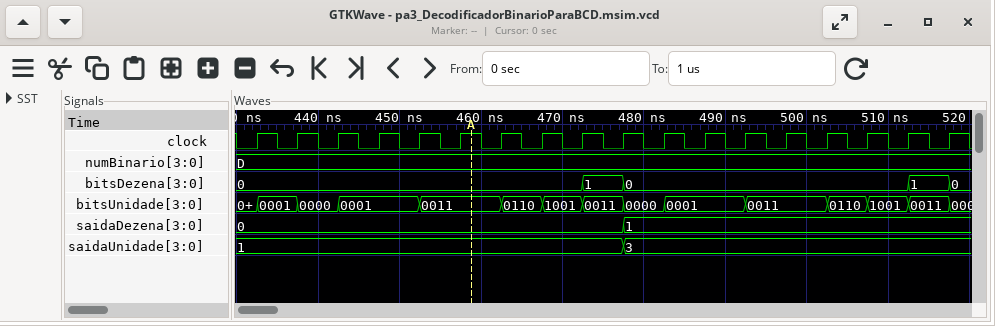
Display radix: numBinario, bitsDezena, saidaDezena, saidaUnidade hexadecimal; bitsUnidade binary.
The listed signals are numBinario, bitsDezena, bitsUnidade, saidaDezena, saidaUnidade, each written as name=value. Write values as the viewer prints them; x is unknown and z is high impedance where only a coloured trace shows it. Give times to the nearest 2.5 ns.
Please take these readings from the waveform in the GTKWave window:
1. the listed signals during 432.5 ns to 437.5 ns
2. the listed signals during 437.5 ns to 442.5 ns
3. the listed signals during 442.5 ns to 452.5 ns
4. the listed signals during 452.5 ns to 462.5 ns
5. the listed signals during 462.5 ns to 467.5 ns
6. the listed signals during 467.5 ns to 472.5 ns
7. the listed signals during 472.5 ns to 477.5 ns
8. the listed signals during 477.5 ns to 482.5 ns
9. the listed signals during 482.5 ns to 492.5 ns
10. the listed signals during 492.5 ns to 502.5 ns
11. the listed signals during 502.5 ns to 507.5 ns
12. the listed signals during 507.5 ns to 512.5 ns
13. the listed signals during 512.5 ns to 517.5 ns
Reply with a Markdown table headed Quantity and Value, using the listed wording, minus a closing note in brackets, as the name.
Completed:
| Quantity | Value |
|---|---|
| the listed signals during 432.5 ns to 437.5 ns | numBinario=D, bitsDezena=0, bitsUnidade=0001, saidaDezena=0, saidaUnidade=1 |
| the listed signals during 437.5 ns to 442.5 ns | numBinario=D, bitsDezena=0, bitsUnidade=0000, saidaDezena=0, saidaUnidade=1 |
| the listed signals during 442.5 ns to 452.5 ns | numBinario=D, bitsDezena=0, bitsUnidade=0001, saidaDezena=0, saidaUnidade=1 |
| the listed signals during 452.5 ns to 462.5 ns | numBinario=D, bitsDezena=0, bitsUnidade=0011, saidaDezena=0, saidaUnidade=1 |
| the listed signals during 462.5 ns to 467.5 ns | numBinario=D, bitsDezena=0, bitsUnidade=0110, saidaDezena=0, saidaUnidade=1 |
| the listed signals during 467.5 ns to 472.5 ns | numBinario=D, bitsDezena=0, bitsUnidade=1001, saidaDezena=0, saidaUnidade=1 |
| the listed signals during 472.5 ns to 477.5 ns | numBinario=D, bitsDezena=1, bitsUnidade=0011, saidaDezena=0, saidaUnidade=1 |
| the listed signals during 477.5 ns to 482.5 ns | numBinario=D, bitsDezena=0, bitsUnidade=0000, saidaDezena=1, saidaUnidade=3 |
| the listed signals during 482.5 ns to 492.5 ns | numBinario=D, bitsDezena=0, bitsUnidade=0001, saidaDezena=1, saidaUnidade=3 |
| the listed signals during 492.5 ns to 502.5 ns | numBinario=D, bitsDezena=0, bitsUnidade=0011, saidaDezena=1, saidaUnidade=3 |
| the listed signals during 502.5 ns to 507.5 ns | numBinario=D, bitsDezena=0, bitsUnidade=0110, saidaDezena=1, saidaUnidade=3 |
| the listed signals during 507.5 ns to 512.5 ns | numBinario=D, bitsDezena=0, bitsUnidade=1001, saidaDezena=1, saidaUnidade=3 |
| the listed signals during 512.5 ns to 517.5 ns | numBinario=D, bitsDezena=1, bitsUnidade=0011, saidaDezena=1, saidaUnidade=3 |
